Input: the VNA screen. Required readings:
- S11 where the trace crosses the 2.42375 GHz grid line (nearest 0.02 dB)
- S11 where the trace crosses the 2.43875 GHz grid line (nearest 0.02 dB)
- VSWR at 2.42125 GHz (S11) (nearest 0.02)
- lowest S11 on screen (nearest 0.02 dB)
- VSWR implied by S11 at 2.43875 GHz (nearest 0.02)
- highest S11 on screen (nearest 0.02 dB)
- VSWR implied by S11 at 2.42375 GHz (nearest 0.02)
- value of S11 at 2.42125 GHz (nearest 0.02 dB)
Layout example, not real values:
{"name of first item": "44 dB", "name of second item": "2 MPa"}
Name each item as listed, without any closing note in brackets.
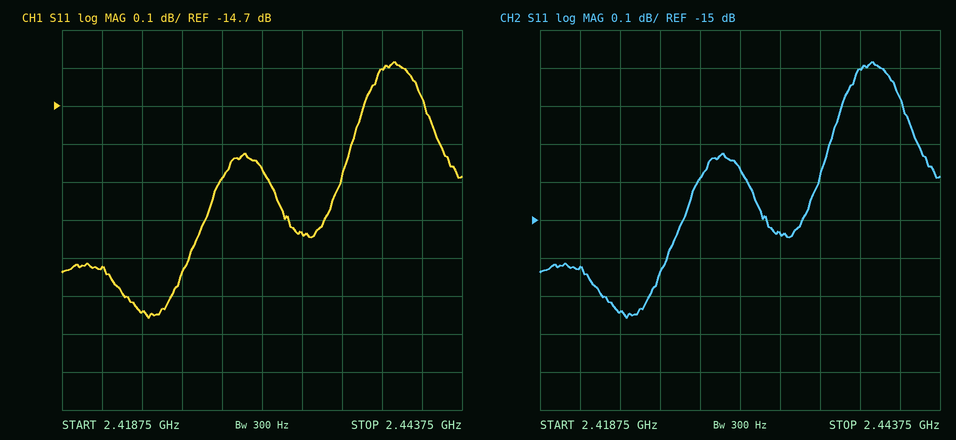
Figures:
{"S11 where the trace crosses the 2.42375 GHz grid line": "-15.24 dB", "S11 where the trace crosses the 2.43875 GHz grid line": "-14.60 dB", "VSWR at 2.42125 GHz (S11)": "1.42", "lowest S11 on screen": "-15.26 dB", "VSWR implied by S11 at 2.43875 GHz": "1.46", "highest S11 on screen": "-14.58 dB", "VSWR implied by S11 at 2.42375 GHz": "1.42", "value of S11 at 2.42125 GHz": "-15.12 dB"}
